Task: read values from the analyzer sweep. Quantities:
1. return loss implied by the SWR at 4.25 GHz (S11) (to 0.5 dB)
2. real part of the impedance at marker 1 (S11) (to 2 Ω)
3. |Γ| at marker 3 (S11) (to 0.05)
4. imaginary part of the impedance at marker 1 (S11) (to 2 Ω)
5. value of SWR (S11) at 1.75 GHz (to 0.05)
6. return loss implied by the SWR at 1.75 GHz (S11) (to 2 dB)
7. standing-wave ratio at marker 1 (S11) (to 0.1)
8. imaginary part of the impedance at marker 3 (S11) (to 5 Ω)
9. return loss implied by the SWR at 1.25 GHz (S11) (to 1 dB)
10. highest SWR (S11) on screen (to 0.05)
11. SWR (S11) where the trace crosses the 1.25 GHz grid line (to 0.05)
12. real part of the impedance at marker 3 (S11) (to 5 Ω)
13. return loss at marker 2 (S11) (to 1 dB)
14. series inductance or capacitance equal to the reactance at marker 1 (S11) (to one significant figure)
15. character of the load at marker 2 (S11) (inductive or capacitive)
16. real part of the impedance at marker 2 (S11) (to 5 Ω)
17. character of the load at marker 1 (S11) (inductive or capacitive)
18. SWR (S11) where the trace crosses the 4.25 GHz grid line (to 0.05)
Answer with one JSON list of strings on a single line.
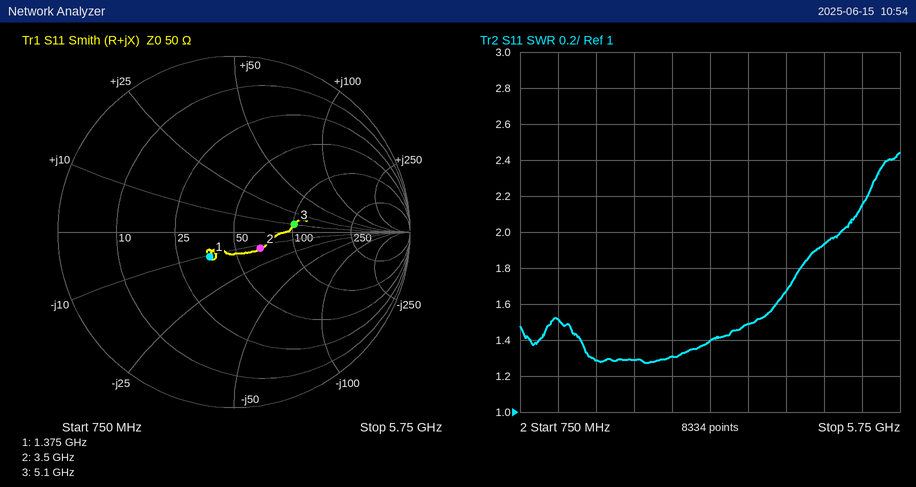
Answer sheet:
["12.0 dB", "36 Ω", "0.35", "-10 Ω", "1.30", "18 dB", "1.5", "+10 Ω", "14 dB", "2.45", "1.50", "100 Ω", "15 dB", "10 pF", "capacitive", "65 Ω", "capacitive", "1.65"]
